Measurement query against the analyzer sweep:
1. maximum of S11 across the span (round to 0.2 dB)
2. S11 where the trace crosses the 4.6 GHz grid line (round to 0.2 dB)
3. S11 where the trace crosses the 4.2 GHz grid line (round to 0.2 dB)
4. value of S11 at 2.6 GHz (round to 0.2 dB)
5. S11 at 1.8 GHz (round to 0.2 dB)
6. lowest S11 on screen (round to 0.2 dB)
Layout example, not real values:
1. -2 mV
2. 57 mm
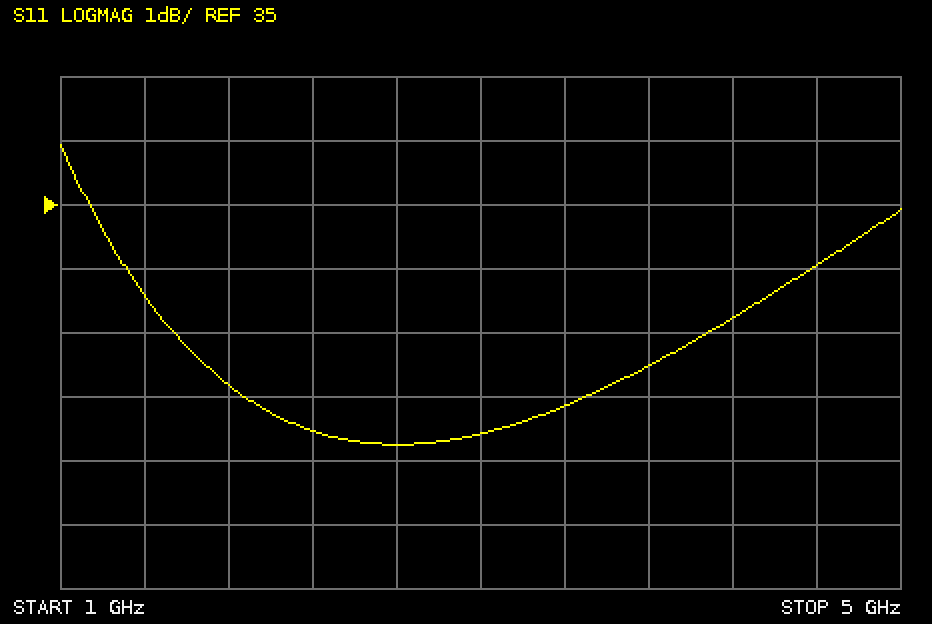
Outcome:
1. 36.0 dB
2. 34.0 dB
3. 33.2 dB
4. 31.2 dB
5. 32.2 dB
6. 31.2 dB
